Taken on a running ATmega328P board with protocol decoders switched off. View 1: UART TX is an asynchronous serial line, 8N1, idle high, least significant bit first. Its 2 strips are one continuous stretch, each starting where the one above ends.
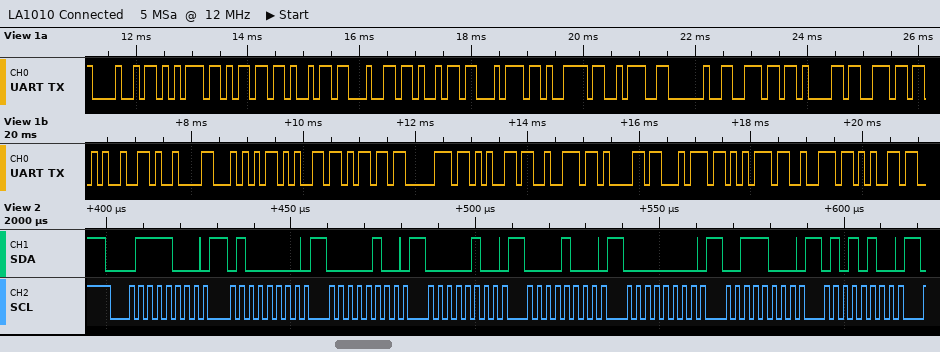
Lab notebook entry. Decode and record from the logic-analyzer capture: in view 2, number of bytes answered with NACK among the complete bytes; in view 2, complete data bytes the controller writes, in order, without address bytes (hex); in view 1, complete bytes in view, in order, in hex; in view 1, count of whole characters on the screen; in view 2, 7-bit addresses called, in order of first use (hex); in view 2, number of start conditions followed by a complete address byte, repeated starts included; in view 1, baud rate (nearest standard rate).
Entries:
0
40 04 04 08 00 38 54
48 75 6D 69 64 69 74 79 3A 20 6E 61 6E 25 09 54 65 6D 70 65 72 61 74 75 72 65
26
0x3C
1
9600 baud
